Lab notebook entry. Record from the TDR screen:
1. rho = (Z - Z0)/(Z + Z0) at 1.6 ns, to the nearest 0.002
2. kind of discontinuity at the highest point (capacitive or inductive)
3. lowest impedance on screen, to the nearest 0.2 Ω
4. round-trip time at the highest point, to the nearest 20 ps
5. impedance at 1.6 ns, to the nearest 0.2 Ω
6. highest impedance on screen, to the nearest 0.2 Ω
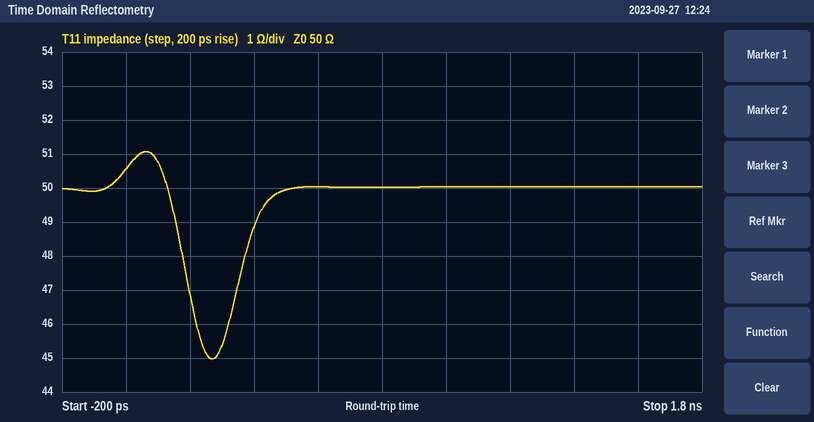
0.000
inductive
45.0 Ω
60 ps
50.0 Ω
51.0 Ω
